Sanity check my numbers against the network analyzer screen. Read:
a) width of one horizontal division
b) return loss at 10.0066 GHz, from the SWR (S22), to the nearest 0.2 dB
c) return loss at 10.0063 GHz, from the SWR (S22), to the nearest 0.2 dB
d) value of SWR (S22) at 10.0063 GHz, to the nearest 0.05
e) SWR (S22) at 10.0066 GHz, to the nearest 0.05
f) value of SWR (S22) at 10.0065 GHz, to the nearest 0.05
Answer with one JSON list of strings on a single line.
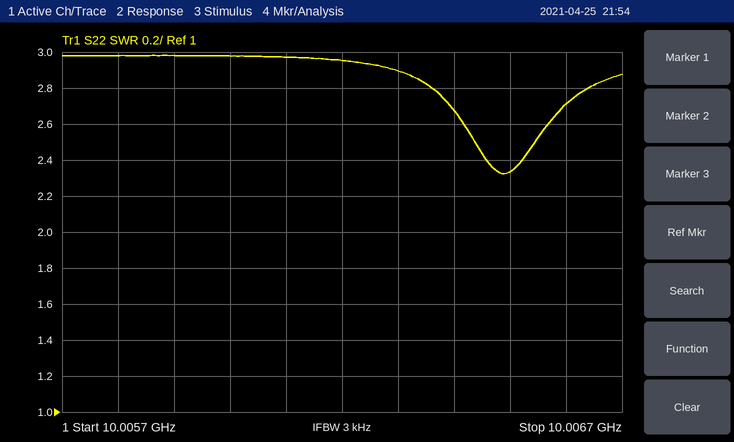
["100 kHz", "6.8 dB", "6.2 dB", "2.90", "2.70", "2.35"]
